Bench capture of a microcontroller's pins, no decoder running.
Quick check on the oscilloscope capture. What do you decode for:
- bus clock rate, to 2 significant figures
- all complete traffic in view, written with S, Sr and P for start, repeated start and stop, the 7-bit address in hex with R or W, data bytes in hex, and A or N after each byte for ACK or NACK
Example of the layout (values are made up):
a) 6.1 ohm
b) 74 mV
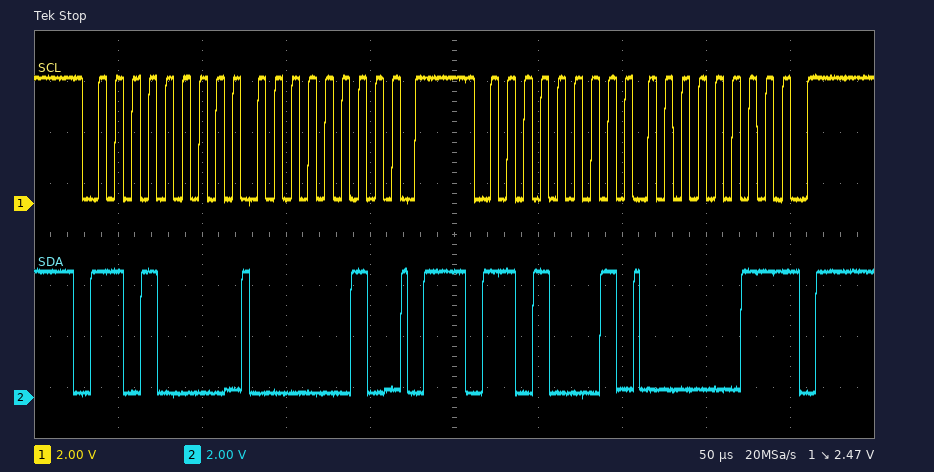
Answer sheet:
a) 100 kHz
b) S 68W A 02 A P S 68R A 03 N P
